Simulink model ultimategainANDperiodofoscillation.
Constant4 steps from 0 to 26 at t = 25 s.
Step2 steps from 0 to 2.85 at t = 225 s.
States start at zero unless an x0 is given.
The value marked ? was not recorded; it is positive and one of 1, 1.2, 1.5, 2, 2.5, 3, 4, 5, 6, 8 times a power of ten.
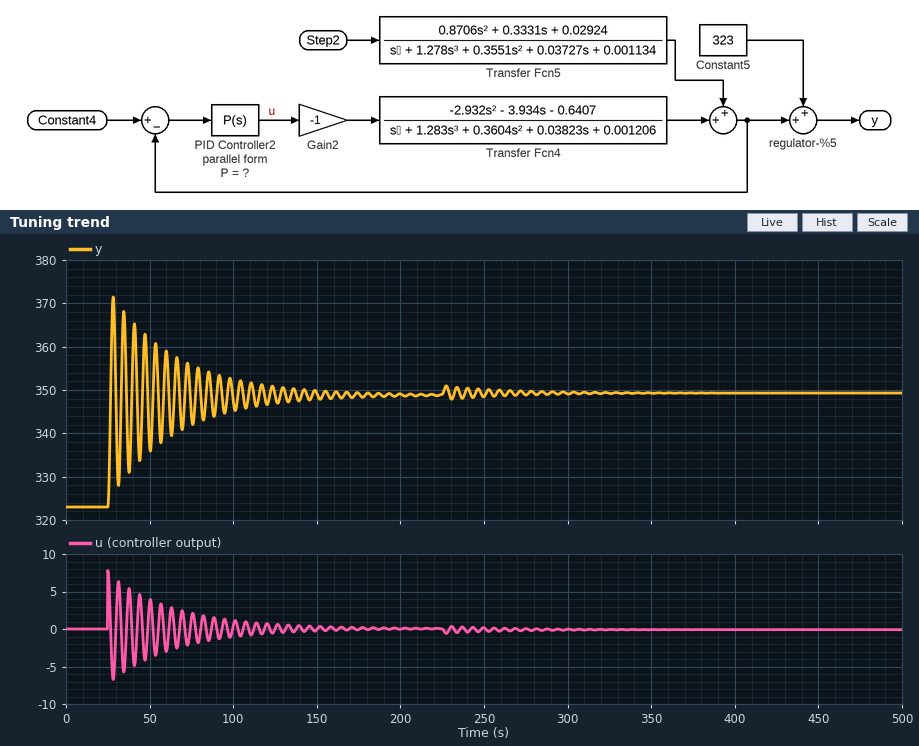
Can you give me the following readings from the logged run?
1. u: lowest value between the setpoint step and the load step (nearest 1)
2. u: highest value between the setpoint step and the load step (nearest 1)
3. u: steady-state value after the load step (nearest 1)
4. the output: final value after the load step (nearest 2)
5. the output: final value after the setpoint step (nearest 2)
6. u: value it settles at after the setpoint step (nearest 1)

-7
8
0
350
348
0
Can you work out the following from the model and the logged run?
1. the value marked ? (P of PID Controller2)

0.3
